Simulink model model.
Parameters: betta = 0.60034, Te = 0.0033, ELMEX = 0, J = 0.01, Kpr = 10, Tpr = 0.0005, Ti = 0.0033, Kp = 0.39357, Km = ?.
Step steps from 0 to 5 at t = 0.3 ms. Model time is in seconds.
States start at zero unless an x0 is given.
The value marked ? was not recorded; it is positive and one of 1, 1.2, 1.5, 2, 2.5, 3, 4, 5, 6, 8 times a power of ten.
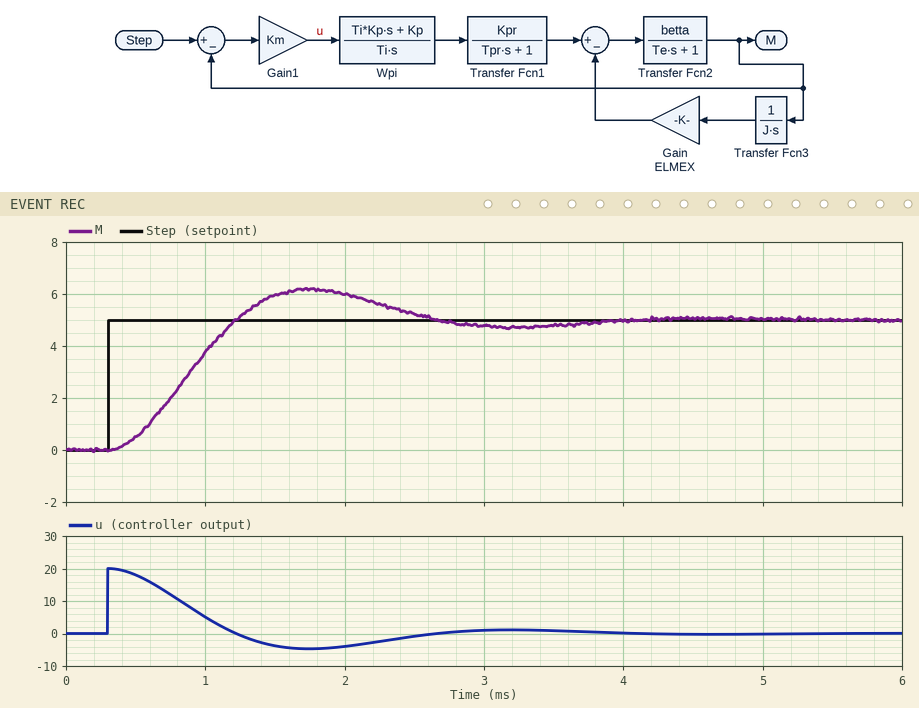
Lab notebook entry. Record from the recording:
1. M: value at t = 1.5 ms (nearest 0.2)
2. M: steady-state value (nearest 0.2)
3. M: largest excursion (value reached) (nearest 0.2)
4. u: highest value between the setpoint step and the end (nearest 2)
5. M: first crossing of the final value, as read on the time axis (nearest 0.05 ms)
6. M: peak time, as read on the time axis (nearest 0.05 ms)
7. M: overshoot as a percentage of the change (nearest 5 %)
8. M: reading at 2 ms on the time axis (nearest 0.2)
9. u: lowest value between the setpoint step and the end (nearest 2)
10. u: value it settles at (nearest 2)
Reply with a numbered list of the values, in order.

1. 6.0
2. 5.0
3. 6.2
4. 20
5. 1.20 ms
6. 1.75 ms
7. 25 %
8. 6.0
9. -4
10. 0
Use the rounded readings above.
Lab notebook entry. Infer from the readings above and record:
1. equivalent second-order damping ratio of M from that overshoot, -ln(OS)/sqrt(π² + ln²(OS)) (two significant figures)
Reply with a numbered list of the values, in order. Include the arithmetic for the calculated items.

1. ln(0.25) = -1.386; 1.386 / sqrt(9.870 + 1.922) = 0.40
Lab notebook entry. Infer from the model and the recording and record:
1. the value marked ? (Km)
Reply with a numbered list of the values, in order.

1. 4
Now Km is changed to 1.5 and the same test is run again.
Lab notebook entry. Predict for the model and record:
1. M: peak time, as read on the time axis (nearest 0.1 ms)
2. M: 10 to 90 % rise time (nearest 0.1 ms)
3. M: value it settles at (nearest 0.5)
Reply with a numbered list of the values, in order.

1. 3.2 ms
2. 1.4 ms
3. 5.0
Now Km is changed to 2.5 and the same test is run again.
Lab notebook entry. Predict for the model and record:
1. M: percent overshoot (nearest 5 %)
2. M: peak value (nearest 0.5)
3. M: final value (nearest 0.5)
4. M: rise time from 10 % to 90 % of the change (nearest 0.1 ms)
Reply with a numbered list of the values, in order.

1. 15 %
2. 5.5
3. 5.0
4. 0.9 ms
